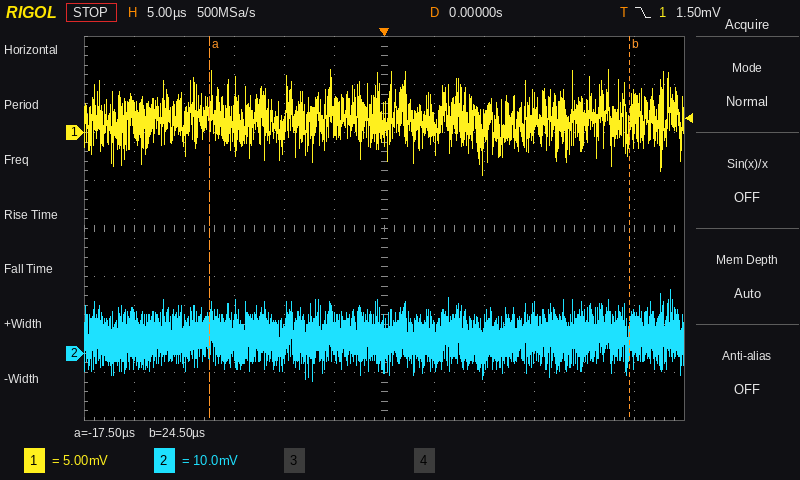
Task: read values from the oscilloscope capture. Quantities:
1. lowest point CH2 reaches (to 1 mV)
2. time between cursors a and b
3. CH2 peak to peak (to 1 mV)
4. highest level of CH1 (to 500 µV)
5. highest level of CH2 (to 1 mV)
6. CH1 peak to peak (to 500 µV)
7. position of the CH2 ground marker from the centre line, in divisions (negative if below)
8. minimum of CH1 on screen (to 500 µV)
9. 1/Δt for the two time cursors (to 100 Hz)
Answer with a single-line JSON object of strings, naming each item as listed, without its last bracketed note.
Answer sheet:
{"lowest point CH2 reaches": "-6 mV", "time between cursors a and b": "42.0 µs", "CH2 peak to peak": "19 mV", "highest level of CH1": "6.5 mV", "highest level of CH2": "13 mV", "CH1 peak to peak": "11.0 mV", "position of the CH2 ground marker from the centre line, in divisions": "-2.6 div", "minimum of CH1 on screen": "-4.5 mV", "1/Δt for the two time cursors": "23.8 kHz"}
